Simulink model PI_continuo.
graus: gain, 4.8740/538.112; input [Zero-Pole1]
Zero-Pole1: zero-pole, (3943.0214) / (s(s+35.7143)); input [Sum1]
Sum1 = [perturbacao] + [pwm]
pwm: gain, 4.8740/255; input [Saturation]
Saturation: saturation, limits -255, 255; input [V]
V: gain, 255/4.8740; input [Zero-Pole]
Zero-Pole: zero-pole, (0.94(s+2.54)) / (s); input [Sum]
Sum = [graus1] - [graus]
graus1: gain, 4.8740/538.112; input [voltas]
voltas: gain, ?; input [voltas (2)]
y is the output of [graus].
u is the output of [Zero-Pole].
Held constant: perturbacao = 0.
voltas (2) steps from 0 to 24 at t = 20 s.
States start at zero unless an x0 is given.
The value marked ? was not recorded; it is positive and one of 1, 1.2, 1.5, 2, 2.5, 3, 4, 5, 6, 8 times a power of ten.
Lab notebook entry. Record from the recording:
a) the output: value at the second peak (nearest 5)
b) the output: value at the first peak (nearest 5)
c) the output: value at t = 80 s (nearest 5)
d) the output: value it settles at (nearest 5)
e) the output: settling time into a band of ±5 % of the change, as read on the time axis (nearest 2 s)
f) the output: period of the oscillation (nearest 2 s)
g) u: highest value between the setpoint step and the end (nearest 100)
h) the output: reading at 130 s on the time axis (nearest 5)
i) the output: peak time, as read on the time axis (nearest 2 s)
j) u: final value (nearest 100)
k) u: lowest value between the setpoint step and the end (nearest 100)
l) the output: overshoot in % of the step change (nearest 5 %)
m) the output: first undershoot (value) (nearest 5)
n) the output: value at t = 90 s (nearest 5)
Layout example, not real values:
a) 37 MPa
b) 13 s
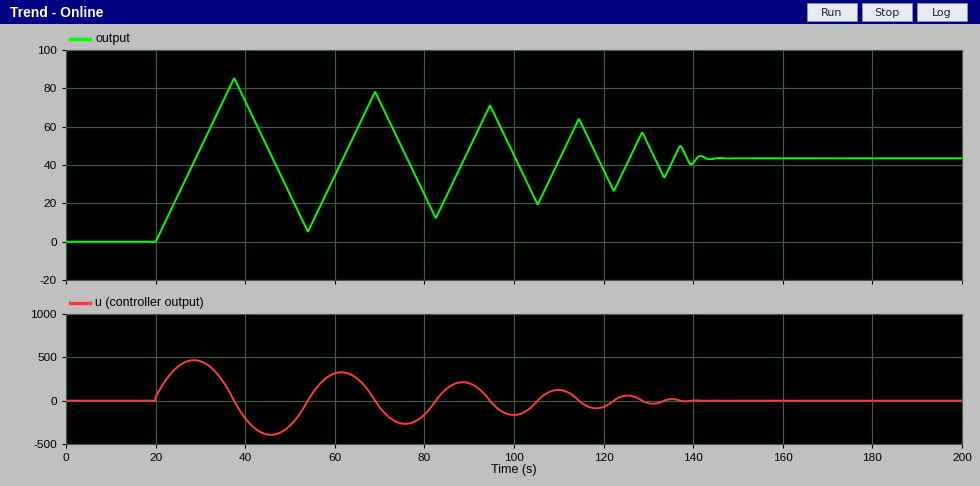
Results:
a) 80
b) 85
c) 25
d) 45
e) 140 s
f) 32 s
g) 500
h) 50
i) 38 s
j) 0
k) -400
l) 95 %
m) 5
n) 50
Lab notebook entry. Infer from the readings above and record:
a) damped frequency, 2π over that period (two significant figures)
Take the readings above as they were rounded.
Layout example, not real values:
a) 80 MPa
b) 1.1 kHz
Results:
a) 0.20 rad/s
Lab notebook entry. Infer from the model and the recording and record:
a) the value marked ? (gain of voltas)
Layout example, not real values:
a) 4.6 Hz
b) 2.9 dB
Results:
a) 200
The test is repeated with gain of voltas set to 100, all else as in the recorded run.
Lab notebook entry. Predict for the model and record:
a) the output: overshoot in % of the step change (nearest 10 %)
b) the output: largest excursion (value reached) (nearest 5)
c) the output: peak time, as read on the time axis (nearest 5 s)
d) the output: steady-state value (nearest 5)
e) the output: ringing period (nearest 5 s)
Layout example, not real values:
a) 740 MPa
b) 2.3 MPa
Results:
a) 90 %
b) 40
c) 30 s
d) 20
e) 15 s
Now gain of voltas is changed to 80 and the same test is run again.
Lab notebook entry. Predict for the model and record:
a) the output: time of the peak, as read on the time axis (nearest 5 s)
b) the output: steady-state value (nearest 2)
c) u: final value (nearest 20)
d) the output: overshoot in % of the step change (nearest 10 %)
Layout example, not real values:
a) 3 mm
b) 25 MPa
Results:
a) 25 s
b) 18
c) 0
d) 90 %
